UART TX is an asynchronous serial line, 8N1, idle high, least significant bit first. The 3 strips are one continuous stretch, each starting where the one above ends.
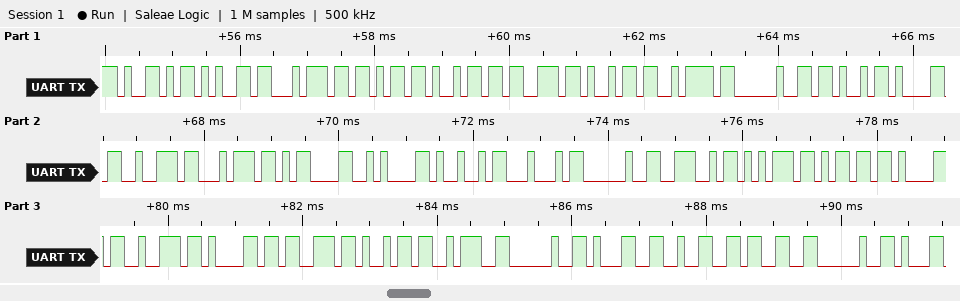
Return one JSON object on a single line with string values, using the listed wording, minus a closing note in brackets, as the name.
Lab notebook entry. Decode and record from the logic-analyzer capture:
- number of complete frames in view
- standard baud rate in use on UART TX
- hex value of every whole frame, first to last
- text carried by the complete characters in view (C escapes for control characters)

{"number of complete frames in view": "32", "standard baud rate in use on UART TX": "9600 baud", "hex value of every whole frame, first to last": "59 65 74 6B 69 73 69 7A 20 4B 61 72 74 0D 0A 49 44 20 4E 75 6D 61 72 61 73 69 3A 20 31 32 33 20", "text carried by the complete characters in view": "\"Yetkisiz Kart\\r\\nID Numarasi: 123 \""}
